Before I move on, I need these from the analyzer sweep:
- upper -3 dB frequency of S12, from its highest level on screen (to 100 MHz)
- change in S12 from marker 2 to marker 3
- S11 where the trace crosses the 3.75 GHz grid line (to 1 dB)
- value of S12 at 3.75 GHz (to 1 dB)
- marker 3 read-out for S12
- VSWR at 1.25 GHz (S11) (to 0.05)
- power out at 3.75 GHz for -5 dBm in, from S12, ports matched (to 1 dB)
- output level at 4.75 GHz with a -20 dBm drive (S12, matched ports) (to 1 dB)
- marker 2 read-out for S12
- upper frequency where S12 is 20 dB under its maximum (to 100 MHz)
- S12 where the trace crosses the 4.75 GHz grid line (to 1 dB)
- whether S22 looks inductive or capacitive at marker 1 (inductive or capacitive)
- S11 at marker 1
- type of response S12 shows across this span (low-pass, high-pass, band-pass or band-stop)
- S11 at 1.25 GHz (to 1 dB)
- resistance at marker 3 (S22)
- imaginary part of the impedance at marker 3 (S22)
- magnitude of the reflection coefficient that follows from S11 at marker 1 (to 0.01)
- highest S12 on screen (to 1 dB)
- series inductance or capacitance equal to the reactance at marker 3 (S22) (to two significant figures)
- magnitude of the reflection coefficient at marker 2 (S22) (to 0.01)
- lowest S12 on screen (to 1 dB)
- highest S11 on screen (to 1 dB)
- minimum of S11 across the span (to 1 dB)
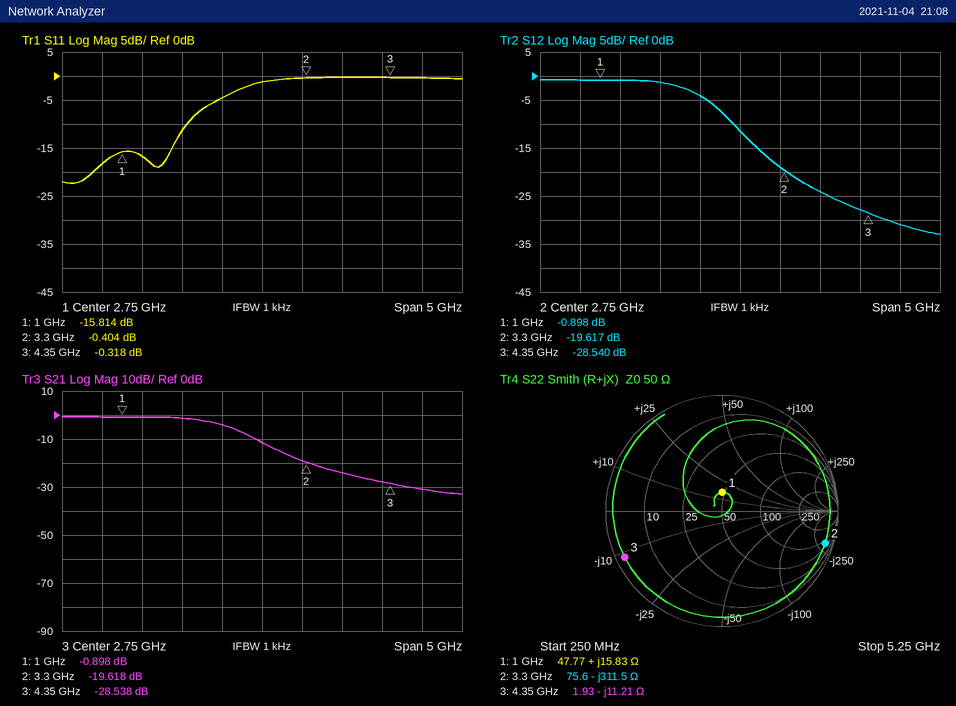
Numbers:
2.2 GHz
-8.923 dB
0 dB
-24 dB
-28.540 dB
1.35
-29 dBm
-51 dBm
-19.617 dB
3.4 GHz
-31 dB
inductive
-15.814 dB
low-pass
-17 dB
1.93 Ω
-11.21 Ω
0.16
-1 dB
3.3 pF
0.93
-33 dB
0 dB
-22 dB
